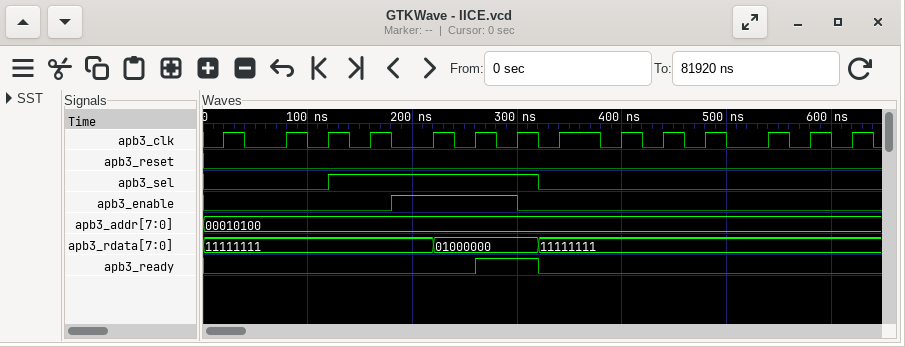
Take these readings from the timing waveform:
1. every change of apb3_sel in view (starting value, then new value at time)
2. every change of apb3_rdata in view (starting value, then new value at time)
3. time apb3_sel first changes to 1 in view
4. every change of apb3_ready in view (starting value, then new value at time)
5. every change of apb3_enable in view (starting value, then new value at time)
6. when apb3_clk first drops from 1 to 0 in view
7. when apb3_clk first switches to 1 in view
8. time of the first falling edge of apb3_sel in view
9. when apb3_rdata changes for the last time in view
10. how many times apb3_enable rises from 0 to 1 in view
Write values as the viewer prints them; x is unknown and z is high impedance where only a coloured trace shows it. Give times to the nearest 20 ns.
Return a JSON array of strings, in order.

["0, 1 at 120 ns, 0 at 320 ns", "11111111, 01000000 at 220 ns, 11111111 at 320 ns", "120 ns", "0, 1 at 260 ns, 0 at 320 ns", "0, 1 at 180 ns, 0 at 300 ns", "40 ns", "20 ns", "320 ns", "320 ns", "1"]
